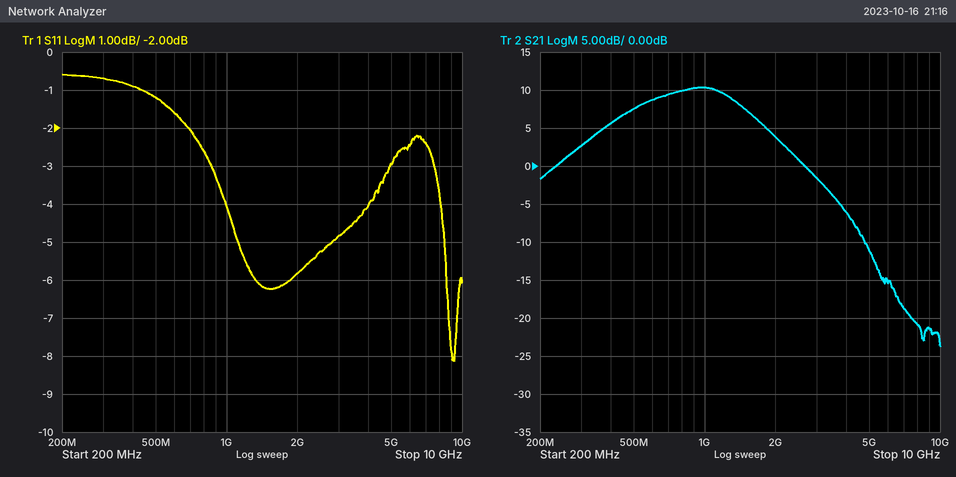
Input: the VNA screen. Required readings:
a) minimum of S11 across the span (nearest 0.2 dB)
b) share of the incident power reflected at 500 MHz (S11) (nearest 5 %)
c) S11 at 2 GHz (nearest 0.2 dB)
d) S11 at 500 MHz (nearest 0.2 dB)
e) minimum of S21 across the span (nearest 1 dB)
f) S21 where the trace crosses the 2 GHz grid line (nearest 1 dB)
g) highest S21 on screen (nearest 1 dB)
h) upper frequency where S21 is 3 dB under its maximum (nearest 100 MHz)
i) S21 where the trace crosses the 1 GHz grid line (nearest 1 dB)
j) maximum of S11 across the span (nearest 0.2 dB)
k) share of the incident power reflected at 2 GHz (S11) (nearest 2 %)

-8.2 dB
75 %
-5.8 dB
-1.2 dB
-24 dB
4 dB
10 dB
1.5 GHz
10 dB
-0.6 dB
26 %
